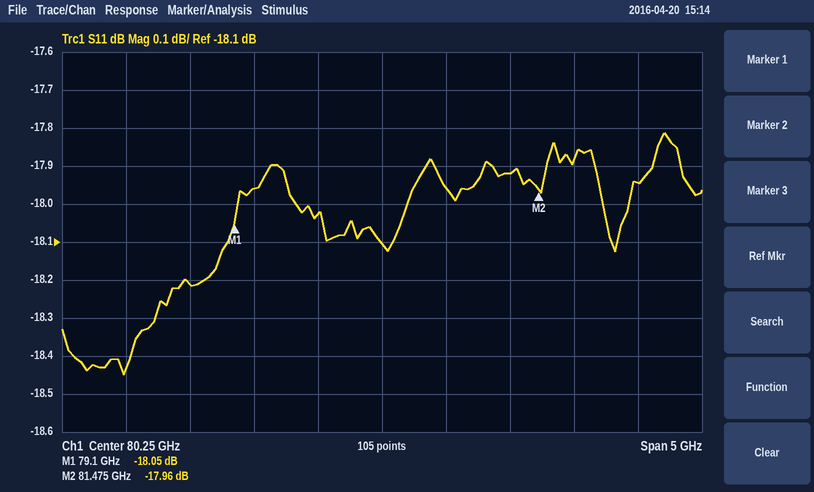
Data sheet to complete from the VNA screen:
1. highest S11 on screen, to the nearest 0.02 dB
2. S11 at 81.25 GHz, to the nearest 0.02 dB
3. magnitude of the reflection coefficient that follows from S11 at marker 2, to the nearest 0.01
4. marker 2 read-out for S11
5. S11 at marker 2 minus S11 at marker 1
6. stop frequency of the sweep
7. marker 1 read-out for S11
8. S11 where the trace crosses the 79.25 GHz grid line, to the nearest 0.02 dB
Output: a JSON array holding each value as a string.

["-17.82 dB", "-17.92 dB", "0.13", "-17.96 dB", "0.09 dB", "82.75 GHz", "-18.05 dB", "-17.96 dB"]
